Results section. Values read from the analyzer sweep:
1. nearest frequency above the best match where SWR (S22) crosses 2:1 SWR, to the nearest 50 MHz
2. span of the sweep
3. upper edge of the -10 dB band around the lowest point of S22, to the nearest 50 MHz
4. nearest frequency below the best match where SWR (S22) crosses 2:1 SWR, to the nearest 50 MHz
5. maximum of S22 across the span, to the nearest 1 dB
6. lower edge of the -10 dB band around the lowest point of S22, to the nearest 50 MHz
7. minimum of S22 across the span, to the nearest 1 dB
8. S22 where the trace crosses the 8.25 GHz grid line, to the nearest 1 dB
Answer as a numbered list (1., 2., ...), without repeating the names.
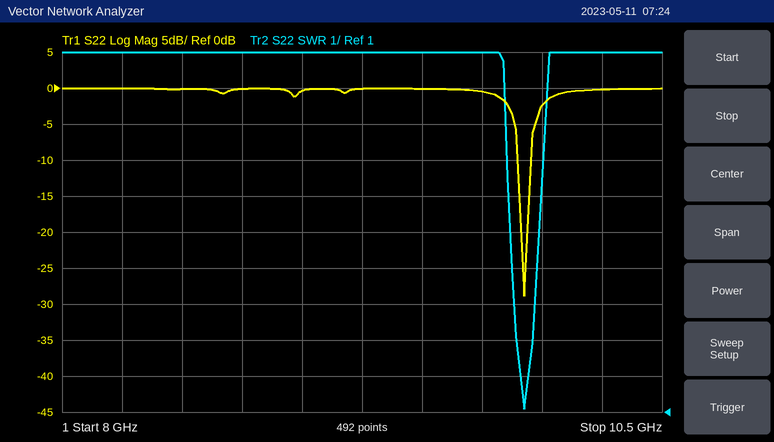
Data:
1. 9.95 GHz
2. 2.5 GHz
3. 9.95 GHz
4. 9.90 GHz
5. 0 dB
6. 9.90 GHz
7. -29 dB
8. 0 dB
